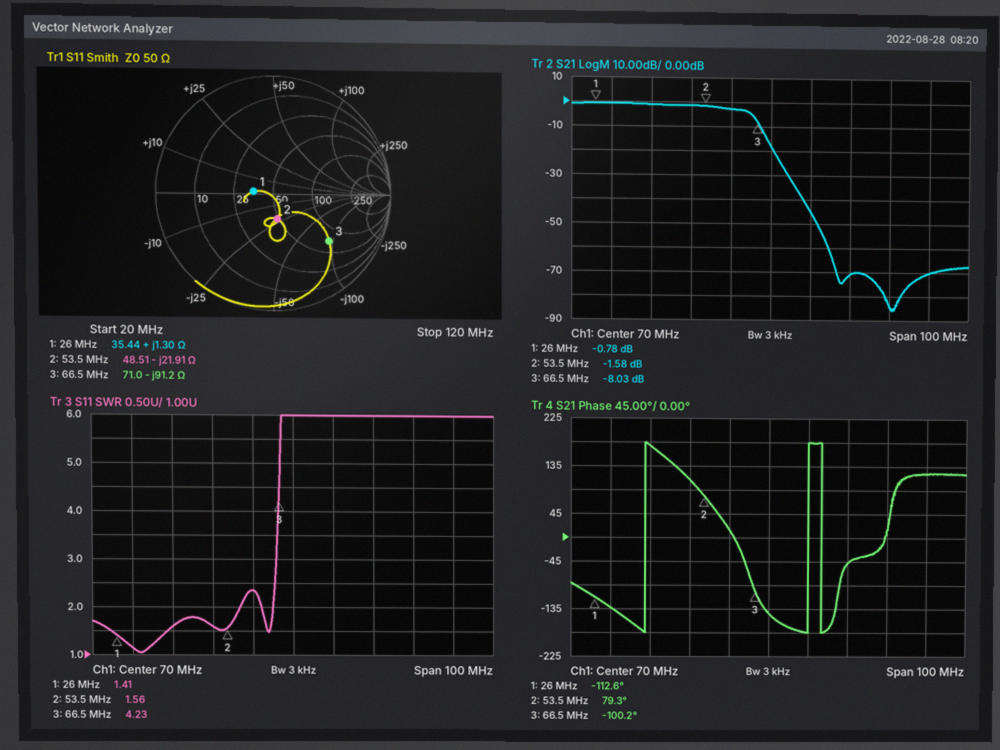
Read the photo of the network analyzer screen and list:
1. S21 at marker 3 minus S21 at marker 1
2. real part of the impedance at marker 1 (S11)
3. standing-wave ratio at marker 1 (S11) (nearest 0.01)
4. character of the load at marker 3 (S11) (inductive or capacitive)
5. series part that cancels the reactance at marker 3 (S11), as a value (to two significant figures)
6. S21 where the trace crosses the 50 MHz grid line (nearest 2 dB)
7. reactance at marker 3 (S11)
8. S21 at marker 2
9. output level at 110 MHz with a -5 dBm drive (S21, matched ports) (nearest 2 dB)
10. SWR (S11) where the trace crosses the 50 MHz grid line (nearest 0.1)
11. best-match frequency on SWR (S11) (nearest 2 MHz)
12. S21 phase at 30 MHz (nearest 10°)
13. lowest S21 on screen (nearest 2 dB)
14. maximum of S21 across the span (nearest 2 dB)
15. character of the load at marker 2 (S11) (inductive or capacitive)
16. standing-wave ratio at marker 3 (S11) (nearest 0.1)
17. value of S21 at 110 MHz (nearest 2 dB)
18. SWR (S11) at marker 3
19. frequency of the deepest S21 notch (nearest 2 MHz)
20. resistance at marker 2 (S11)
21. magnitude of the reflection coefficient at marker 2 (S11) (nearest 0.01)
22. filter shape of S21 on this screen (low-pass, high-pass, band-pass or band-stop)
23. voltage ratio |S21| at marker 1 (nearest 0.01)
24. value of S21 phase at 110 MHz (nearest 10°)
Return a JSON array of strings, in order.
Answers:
["-7.25 dB", "35.44 Ω", "1.41", "capacitive", "220 nH", "-2 dB", "-91.2 Ω", "-1.58 dB", "-76 dBm", "1.6", "32 MHz", "-130°", "-86 dB", "0 dB", "capacitive", "4.2", "-70 dB", "4.23", "100 MHz", "48.51 Ω", "0.22", "low-pass", "0.91", "120°"]
